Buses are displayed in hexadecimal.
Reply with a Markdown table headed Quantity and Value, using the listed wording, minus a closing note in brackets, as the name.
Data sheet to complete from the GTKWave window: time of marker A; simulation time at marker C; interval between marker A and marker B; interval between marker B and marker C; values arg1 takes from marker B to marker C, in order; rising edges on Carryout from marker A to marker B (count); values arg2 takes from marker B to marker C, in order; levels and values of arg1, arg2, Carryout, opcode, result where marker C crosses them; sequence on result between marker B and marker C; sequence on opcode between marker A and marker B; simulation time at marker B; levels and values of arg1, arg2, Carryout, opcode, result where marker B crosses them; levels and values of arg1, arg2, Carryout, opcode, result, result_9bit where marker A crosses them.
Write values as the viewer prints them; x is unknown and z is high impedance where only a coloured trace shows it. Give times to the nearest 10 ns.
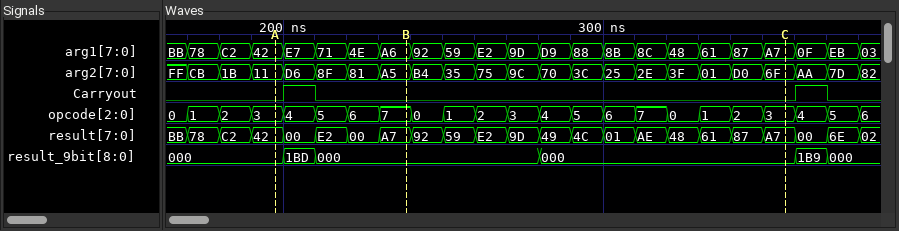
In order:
| Quantity | Value |
|---|---|
| time of marker A | 200 ns |
| simulation time at marker C | 360 ns |
| interval between marker A and marker B | 40 ns |
| interval between marker B and marker C | 120 ns |
| values arg1 takes from marker B to marker C, in order | A6, 92, 59, E2, 9D, D9, 88, 8B, 8C, 48, 61, 87, A7 |
| rising edges on Carryout from marker A to marker B | 1 |
| values arg2 takes from marker B to marker C, in order | A5, B4, 35, 75, 9C, 70, 3C, 25, 2E, 3F, 01, D0, 6F |
| levels and values of arg1, arg2, Carryout, opcode, result where marker C crosses them | arg1=A7, arg2=6F, Carryout=0, opcode=3, result=A7 |
| sequence on result between marker B and marker C | A7, 92, 59, E2, 9D, 49, 4C, 01, AE, 48, 61, 87, A7 |
| sequence on opcode between marker A and marker B | 3, 4, 5, 6, 7 |
| simulation time at marker B | 240 ns |
| levels and values of arg1, arg2, Carryout, opcode, result where marker B crosses them | arg1=A6, arg2=A5, Carryout=0, opcode=7, result=A7 |
| levels and values of arg1, arg2, Carryout, opcode, result, result_9bit where marker A crosses them | arg1=42, arg2=11, Carryout=0, opcode=3, result=42, result_9bit=000 |
